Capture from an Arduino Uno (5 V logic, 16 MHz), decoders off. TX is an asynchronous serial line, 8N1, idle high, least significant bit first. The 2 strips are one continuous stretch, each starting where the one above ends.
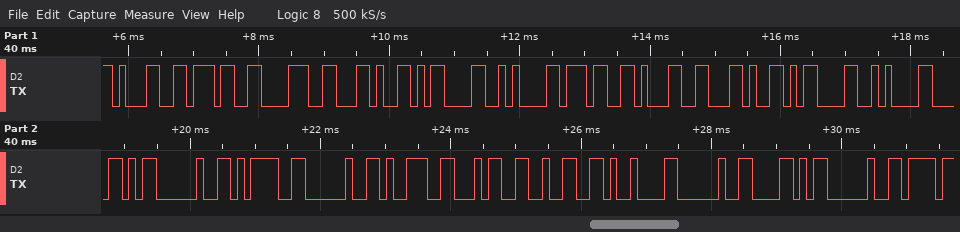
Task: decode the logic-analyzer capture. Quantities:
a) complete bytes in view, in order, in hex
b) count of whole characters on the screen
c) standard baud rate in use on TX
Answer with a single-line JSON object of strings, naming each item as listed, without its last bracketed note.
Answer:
{"complete bytes in view, in order, in hex": "31 37 38 2C 0D 0A 37 31 2C 0D 0A 58 20 3D 20 39 34 32 09 20 58 20", "count of whole characters on the screen": "22", "standard baud rate in use on TX": "9600 baud"}
